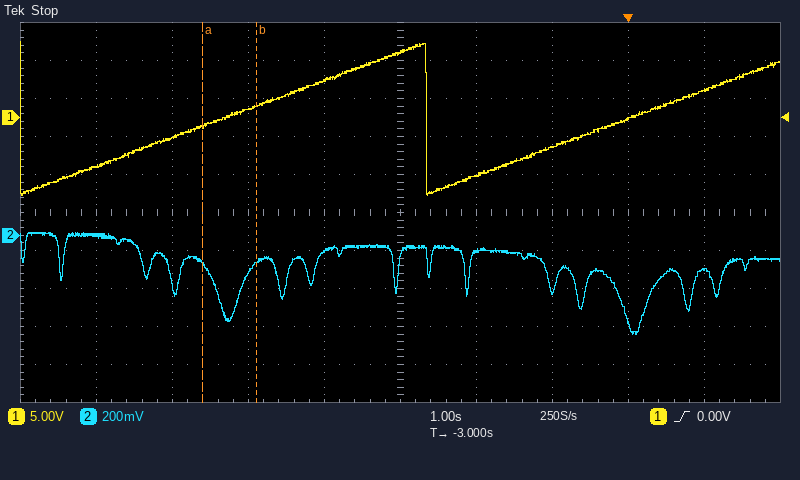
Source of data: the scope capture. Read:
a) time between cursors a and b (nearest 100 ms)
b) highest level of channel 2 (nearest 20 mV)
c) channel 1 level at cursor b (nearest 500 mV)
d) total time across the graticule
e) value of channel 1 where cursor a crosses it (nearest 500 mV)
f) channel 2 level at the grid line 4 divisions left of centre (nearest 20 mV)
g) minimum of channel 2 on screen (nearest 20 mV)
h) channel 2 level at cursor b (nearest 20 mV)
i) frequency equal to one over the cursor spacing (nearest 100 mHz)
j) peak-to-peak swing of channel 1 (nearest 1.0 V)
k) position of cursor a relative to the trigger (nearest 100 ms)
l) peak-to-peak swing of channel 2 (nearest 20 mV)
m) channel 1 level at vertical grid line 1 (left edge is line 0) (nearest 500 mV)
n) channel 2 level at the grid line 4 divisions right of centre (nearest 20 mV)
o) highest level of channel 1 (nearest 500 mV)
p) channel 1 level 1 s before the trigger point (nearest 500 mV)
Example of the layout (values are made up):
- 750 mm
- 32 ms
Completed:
- 700 ms
- 20 mV
- 1.5 V
- 10 s
- -1.0 V
- 0 mV
- -520 mV
- -140 mV
- 1.4 Hz
- 20.0 V
- -5.6 s
- 540 mV
- -6.5 V
- -180 mV
- 10.0 V
- -4.0 V
